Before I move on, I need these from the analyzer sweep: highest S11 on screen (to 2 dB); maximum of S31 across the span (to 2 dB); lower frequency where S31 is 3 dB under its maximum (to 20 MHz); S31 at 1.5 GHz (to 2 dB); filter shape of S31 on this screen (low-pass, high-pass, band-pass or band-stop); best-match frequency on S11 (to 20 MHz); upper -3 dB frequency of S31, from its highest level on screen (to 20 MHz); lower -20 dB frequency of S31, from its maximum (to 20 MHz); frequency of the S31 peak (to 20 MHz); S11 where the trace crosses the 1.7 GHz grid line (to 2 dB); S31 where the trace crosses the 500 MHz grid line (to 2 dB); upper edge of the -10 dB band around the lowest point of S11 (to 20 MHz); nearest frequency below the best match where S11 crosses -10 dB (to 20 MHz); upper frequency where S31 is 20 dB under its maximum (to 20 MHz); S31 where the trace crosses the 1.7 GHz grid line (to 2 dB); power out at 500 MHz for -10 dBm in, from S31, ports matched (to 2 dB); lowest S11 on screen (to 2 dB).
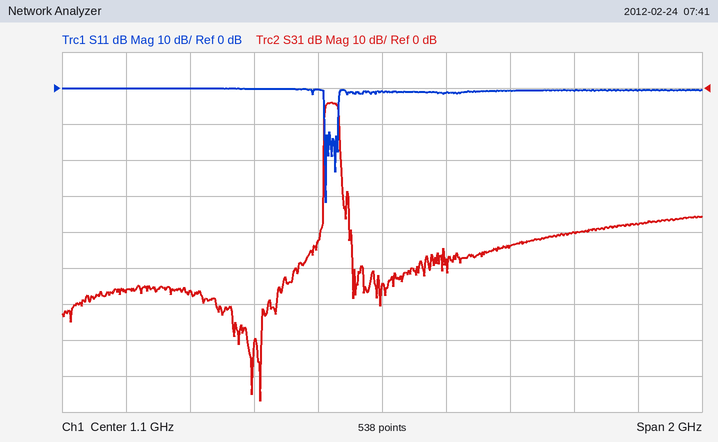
0 dB
-4 dB
920 MHz
-44 dB
band-pass
920 MHz
960 MHz
920 MHz
940 MHz
0 dB
-56 dB
960 MHz
920 MHz
980 MHz
-40 dB
-66 dBm
-32 dB
